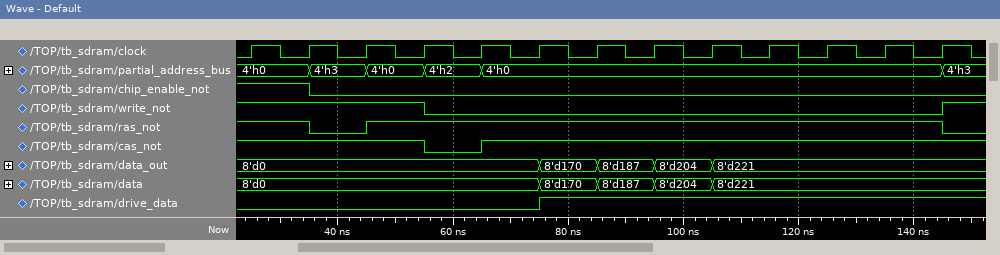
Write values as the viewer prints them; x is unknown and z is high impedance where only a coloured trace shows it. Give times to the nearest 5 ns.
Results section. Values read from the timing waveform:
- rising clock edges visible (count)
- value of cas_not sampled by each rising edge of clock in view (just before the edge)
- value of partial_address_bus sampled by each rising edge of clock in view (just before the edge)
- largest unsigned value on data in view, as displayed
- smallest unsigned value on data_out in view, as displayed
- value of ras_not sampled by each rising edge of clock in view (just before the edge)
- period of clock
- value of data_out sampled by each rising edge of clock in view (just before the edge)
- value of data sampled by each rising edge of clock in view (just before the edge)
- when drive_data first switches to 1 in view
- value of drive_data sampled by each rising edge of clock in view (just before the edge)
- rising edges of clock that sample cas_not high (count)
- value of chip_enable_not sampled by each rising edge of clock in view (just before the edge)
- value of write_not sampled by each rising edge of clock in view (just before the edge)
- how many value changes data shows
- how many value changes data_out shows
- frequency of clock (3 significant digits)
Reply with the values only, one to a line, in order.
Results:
13
1 1 1 1 0 1 1 1 1 1 1 1 1
4'h0, 4'h0, 4'h3, 4'h0, 4'h2, 4'h0, 4'h0, 4'h0, 4'h0, 4'h0, 4'h0, 4'h0, 4'h0
8'd221
8'd0
1 1 0 1 1 1 1 1 1 1 1 1 1
10 ns
8'd0, 8'd0, 8'd0, 8'd0, 8'd0, 8'd0, 8'd170, 8'd187, 8'd204, 8'd221, 8'd221, 8'd221, 8'd221
8'd0, 8'd0, 8'd0, 8'd0, 8'd0, 8'd0, 8'd170, 8'd187, 8'd204, 8'd221, 8'd221, 8'd221, 8'd221
75 ns
0 0 0 0 0 0 1 1 1 1 1 1 1
12
1 1 0 0 0 0 0 0 0 0 0 0 0
1 1 1 1 0 0 0 0 0 0 0 0 0
4
4
100 MHz
